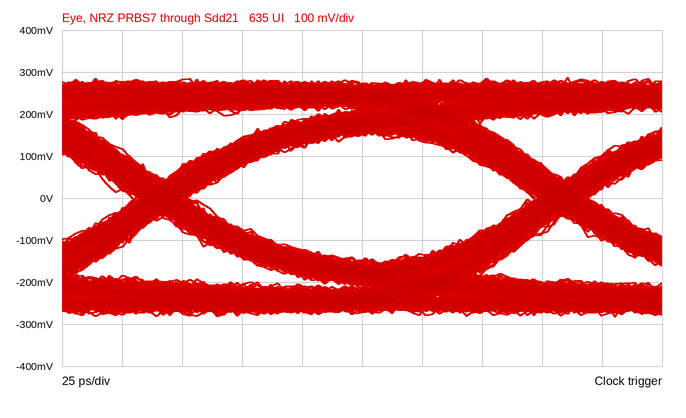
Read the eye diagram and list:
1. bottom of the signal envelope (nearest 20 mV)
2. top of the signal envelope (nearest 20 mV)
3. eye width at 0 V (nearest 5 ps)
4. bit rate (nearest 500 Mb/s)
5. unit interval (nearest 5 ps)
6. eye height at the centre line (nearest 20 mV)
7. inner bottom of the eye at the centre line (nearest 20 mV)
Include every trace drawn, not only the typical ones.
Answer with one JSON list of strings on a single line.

["-280 mV", "280 mV", "145 ps", "6.0 Gb/s", "165 ps", "300 mV", "-140 mV"]
